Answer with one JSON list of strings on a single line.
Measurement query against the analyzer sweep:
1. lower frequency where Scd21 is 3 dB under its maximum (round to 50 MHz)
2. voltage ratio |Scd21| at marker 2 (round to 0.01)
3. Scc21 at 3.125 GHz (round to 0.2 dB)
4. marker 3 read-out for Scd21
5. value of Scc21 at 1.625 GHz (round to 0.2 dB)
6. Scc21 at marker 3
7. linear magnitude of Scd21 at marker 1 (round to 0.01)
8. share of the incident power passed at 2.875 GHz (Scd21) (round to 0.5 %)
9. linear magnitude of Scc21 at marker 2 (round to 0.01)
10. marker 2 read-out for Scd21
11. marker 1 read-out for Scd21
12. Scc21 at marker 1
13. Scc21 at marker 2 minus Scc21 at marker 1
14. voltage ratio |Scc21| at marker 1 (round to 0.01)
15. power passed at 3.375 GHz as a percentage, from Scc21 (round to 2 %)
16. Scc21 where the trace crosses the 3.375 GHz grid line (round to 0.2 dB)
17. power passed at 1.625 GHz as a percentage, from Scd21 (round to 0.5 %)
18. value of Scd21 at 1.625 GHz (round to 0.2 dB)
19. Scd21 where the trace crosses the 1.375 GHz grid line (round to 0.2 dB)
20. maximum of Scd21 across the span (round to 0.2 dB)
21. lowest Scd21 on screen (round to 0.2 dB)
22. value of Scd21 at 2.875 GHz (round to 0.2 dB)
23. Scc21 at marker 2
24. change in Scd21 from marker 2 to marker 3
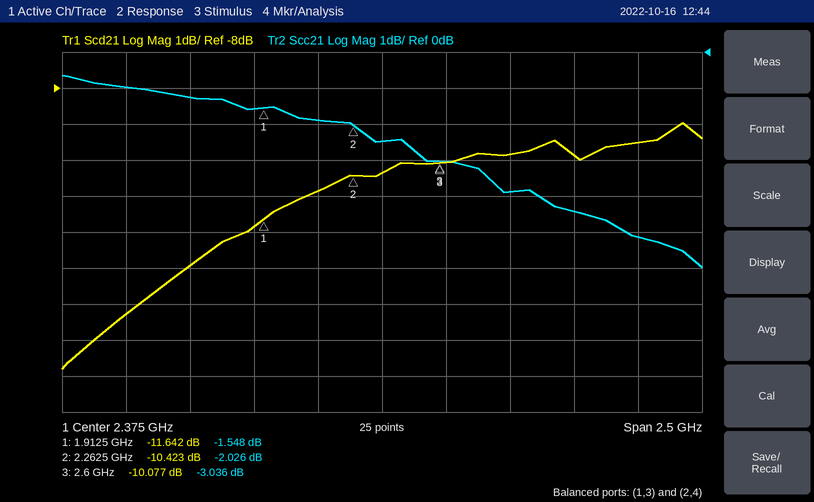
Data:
["1.85 GHz", "0.30", "-4.4 dB", "-10.077 dB", "-1.2 dB", "-3.036 dB", "0.26", "10.5 %", "0.79", "-10.423 dB", "-11.642 dB", "-1.548 dB", "-0.478 dB", "0.84", "30 %", "-5.2 dB", "5.0 %", "-13.0 dB", "-14.2 dB", "-9.0 dB", "-15.8 dB", "-9.8 dB", "-2.026 dB", "0.346 dB"]
